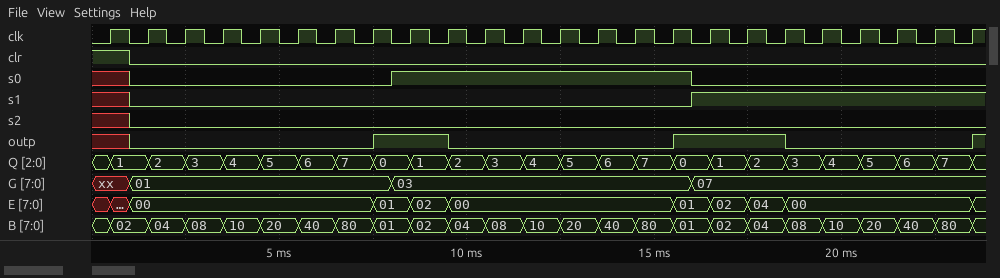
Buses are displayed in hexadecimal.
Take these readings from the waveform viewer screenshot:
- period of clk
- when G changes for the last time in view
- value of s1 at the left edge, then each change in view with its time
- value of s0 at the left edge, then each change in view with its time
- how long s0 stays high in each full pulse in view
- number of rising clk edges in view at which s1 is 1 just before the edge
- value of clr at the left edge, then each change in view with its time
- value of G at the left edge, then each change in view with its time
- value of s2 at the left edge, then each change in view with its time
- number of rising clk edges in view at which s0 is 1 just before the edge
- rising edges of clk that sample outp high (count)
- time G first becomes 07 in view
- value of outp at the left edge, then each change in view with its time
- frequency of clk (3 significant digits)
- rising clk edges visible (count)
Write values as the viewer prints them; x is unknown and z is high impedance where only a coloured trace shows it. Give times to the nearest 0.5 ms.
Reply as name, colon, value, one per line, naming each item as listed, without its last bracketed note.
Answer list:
period of clk: 1 ms
when G changes for the last time in view: 16 ms
value of s1 at the left edge, then each change in view with its time: x, 0 at 1 ms, 1 at 16 ms
value of s0 at the left edge, then each change in view with its time: x, 0 at 1 ms, 1 at 8 ms, 0 at 16 ms
how long s0 stays high in each full pulse in view: 8 ms
number of rising clk edges in view at which s1 is 1 just before the edge: 8
value of clr at the left edge, then each change in view with its time: 1, 0 at 1 ms
value of G at the left edge, then each change in view with its time: xx, 01 at 1 ms, 03 at 8 ms, 07 at 16 ms
value of s2 at the left edge, then each change in view with its time: x, 0 at 1 ms
number of rising clk edges in view at which s0 is 1 just before the edge: 8
rising edges of clk that sample outp high: 5
time G first becomes 07 in view: 16 ms
value of outp at the left edge, then each change in view with its time: x, 0 at 1 ms, 1 at 7.5 ms, 0 at 9.5 ms, 1 at 15.5 ms, 0 at 18.5 ms, 1 at 23.5 ms
frequency of clk: 1.00 kHz
rising clk edges visible: 24
